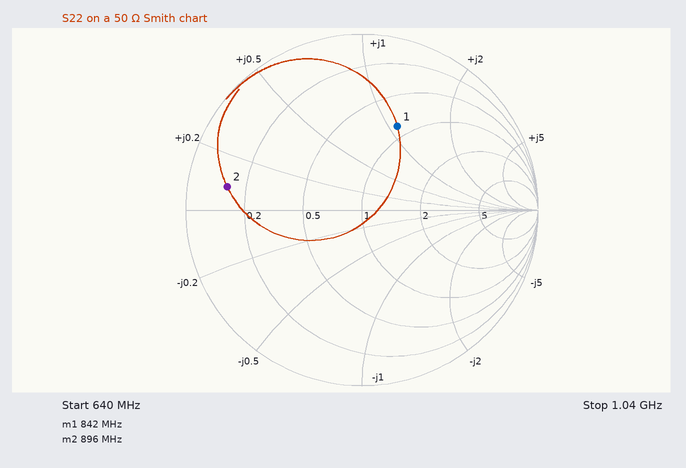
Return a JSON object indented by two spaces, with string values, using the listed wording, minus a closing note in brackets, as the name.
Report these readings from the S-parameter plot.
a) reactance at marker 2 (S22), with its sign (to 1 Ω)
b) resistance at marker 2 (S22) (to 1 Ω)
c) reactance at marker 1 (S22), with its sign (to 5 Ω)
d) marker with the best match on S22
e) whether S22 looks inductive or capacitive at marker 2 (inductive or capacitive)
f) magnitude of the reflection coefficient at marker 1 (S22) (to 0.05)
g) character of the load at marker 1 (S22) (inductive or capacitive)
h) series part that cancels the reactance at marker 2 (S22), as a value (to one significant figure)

{
  "reactance at marker 2 (S22), with its sign": "+4 Ω",
  "resistance at marker 2 (S22)": "6 Ω",
  "reactance at marker 1 (S22), with its sign": "+55 Ω",
  "marker with the best match on S22": "marker 1",
  "whether S22 looks inductive or capacitive at marker 2": "inductive",
  "magnitude of the reflection coefficient at marker 1 (S22)": "0.50",
  "character of the load at marker 1 (S22)": "inductive",
  "series part that cancels the reactance at marker 2 (S22), as a value": "40 pF"
}
